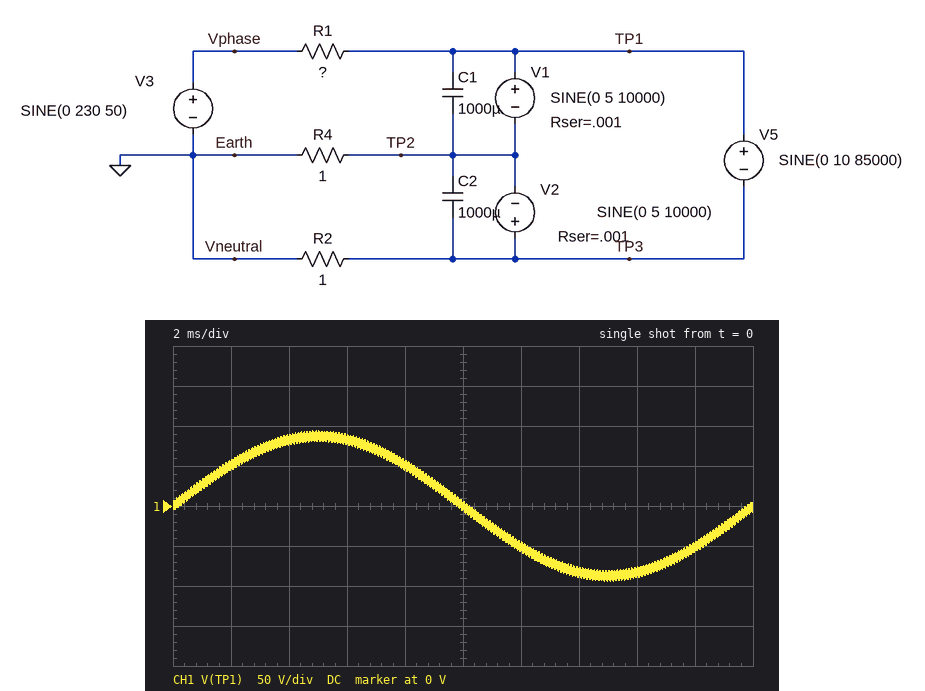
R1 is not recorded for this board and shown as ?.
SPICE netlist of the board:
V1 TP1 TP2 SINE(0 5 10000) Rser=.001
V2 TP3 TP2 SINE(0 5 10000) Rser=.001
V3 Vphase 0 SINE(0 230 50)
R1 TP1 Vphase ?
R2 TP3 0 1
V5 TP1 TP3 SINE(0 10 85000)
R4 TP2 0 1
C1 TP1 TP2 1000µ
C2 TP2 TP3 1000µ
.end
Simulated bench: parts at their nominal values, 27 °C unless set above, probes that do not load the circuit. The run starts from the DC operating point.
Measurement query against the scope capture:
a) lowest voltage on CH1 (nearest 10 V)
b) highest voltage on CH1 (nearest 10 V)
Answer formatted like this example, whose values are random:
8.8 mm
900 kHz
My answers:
-90 V
90 V
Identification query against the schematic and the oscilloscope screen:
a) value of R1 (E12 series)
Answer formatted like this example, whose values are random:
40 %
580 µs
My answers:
0.82 Ω
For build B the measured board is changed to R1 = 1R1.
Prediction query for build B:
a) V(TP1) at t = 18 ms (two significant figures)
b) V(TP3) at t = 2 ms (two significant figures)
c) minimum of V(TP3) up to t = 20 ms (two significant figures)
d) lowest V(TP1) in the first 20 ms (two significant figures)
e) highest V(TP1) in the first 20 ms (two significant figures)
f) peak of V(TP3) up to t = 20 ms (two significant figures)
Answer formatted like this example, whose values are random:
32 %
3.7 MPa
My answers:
-42 V
42 V
-78 V
-79 V
79 V
78 V
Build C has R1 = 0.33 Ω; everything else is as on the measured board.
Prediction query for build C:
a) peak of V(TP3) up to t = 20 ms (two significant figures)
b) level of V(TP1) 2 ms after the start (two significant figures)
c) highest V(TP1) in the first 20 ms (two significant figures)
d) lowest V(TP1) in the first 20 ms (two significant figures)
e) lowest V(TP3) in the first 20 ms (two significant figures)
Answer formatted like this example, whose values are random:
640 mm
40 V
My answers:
150 V
81 V
140 V
-140 V
-150 V
